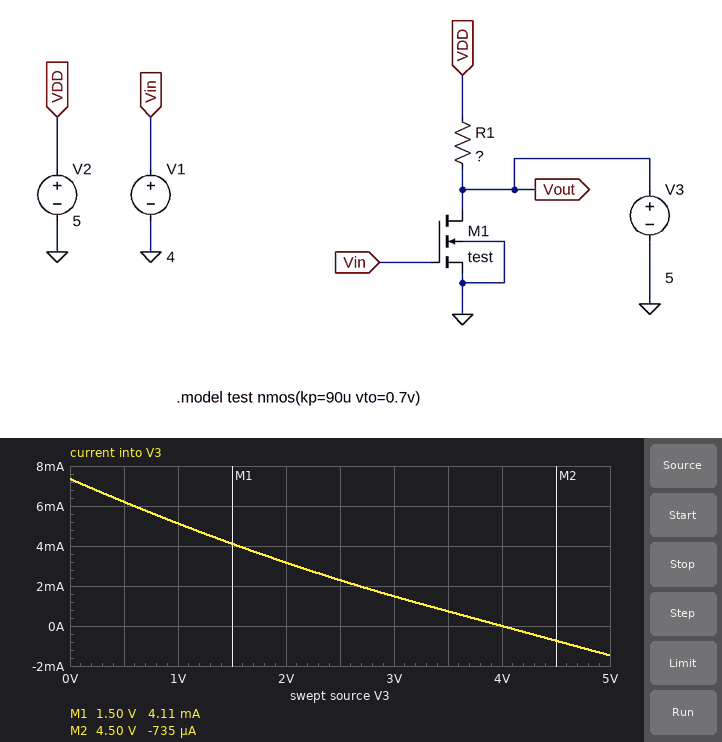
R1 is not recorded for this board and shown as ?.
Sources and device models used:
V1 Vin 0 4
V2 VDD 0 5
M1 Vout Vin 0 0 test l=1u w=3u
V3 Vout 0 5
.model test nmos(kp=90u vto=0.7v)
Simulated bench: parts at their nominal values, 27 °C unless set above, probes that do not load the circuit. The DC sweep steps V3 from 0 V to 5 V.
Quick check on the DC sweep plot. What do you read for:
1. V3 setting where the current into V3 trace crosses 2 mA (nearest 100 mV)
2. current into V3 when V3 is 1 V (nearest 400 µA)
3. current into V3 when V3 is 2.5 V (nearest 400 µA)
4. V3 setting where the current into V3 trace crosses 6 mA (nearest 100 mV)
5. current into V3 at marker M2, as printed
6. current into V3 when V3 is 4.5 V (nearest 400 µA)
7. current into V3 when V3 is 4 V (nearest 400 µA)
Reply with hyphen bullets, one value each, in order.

- 2.7 V
- 5.2 mA
- 2.4 mA
- 600 mV
- -735 µA
- -800 µA
- 0 A
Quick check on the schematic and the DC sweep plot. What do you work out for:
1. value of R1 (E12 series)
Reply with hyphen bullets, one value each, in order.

- 680 Ω
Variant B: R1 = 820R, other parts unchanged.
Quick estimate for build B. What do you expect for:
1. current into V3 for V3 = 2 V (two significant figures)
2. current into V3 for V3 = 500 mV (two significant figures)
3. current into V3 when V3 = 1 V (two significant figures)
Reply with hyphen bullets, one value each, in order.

- 2.4 mA
- 5.1 mA
- 4.1 mA
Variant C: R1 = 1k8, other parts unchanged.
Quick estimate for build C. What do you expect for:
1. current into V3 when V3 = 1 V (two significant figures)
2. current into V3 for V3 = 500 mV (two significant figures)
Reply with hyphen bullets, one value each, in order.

- 1.5 mA
- 2.1 mA
